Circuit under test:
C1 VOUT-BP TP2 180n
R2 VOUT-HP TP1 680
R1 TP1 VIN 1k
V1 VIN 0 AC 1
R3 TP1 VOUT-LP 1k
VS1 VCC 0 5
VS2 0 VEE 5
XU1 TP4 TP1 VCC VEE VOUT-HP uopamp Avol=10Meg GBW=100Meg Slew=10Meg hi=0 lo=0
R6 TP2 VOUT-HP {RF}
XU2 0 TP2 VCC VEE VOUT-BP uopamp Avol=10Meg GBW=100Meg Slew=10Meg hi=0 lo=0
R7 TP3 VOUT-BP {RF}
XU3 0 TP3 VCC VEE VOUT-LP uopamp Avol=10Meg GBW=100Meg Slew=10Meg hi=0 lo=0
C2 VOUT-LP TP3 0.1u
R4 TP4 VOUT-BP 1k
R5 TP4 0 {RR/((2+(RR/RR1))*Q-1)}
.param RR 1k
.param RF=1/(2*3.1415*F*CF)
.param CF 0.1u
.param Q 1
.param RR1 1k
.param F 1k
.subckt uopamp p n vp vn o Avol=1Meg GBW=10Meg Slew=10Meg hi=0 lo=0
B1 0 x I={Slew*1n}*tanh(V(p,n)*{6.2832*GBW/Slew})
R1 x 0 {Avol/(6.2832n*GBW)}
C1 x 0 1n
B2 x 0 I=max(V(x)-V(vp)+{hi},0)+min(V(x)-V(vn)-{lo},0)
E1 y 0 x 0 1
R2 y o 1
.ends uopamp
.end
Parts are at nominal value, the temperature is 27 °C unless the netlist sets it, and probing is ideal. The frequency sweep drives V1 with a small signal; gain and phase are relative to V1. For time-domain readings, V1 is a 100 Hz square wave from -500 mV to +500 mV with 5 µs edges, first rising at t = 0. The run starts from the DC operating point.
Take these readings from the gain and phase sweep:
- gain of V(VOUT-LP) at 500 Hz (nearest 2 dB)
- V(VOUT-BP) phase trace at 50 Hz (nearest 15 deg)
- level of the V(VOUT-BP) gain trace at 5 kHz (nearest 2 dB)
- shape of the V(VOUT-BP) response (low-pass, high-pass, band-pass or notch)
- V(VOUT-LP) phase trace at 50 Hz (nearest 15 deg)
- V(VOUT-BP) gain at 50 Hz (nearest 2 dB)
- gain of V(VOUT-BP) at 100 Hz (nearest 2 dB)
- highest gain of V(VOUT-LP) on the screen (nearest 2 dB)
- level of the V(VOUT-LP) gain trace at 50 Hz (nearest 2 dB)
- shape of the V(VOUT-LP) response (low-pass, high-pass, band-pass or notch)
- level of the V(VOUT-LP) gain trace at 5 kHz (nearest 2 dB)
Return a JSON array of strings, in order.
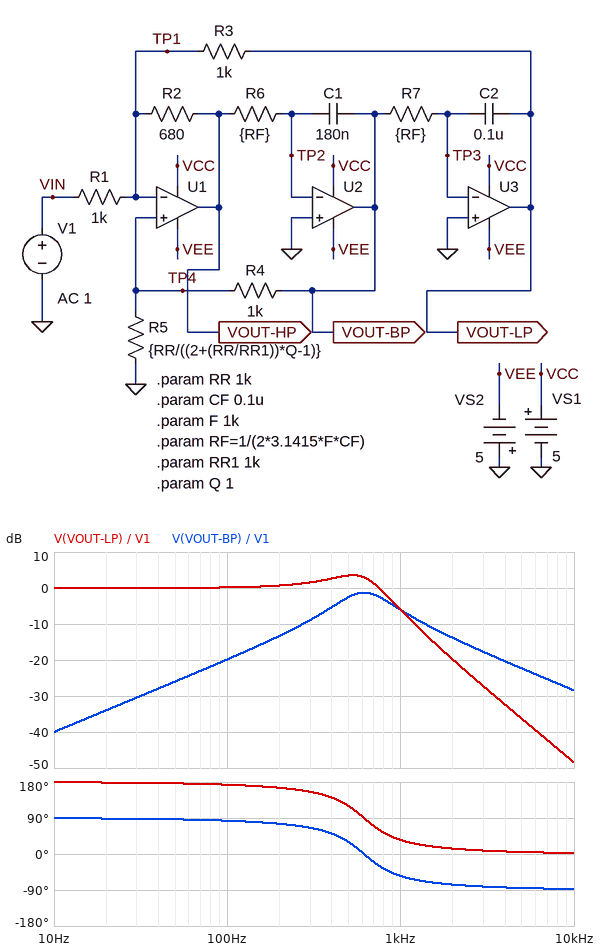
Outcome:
["4 dB", "90 deg", "-22 dB", "band-pass", "180 deg", "-26 dB", "-20 dB", "4 dB", "0 dB", "low-pass", "-36 dB"]
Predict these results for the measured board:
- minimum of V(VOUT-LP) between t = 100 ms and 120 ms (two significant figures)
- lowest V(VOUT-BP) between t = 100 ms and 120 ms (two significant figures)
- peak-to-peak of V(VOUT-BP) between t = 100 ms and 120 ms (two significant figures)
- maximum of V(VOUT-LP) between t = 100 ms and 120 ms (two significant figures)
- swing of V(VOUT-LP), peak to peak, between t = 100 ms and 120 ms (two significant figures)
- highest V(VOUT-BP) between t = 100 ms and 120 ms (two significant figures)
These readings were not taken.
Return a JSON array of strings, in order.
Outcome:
["-800 mV", "-390 mV", "780 mV", "800 mV", "1.6 V", "390 mV"]
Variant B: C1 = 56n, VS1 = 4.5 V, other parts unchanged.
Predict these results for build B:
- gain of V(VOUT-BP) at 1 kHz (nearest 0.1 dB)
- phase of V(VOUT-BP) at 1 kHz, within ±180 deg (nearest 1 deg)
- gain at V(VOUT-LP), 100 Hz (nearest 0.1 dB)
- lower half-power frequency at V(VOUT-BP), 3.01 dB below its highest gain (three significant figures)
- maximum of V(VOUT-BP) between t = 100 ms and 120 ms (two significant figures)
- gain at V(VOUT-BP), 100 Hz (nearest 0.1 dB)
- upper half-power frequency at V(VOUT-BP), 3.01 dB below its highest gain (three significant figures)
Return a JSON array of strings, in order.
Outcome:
["-1.4 dB", "9 deg", "0 dB", "604 Hz", "530 mV", "-20.0 dB", "2.01 kHz"]
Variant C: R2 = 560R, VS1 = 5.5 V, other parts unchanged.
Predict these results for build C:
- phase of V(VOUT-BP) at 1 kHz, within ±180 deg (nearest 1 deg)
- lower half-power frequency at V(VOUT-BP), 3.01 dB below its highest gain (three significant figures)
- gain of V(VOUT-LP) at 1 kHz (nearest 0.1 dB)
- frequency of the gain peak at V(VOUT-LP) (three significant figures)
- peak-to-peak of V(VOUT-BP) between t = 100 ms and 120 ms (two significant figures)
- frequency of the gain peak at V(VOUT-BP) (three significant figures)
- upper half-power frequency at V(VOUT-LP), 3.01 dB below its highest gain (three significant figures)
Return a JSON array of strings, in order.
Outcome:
["-60 deg", "395 Hz", "-8.1 dB", "484 Hz", "710 mV", "558 Hz", "663 Hz"]
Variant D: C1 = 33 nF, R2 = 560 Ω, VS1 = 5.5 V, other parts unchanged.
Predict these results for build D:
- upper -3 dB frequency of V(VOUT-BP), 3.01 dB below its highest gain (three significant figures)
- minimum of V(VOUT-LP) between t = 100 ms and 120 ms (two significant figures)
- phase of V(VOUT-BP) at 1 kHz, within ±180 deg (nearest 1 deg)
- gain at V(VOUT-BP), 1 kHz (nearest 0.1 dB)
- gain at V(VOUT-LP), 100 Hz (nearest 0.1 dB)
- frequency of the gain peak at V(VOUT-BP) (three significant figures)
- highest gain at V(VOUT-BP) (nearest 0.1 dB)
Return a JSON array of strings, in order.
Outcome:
["2.76 kHz", "-510 mV", "18 deg", "-2.5 dB", "0 dB", "1.30 kHz", "-2.0 dB"]
